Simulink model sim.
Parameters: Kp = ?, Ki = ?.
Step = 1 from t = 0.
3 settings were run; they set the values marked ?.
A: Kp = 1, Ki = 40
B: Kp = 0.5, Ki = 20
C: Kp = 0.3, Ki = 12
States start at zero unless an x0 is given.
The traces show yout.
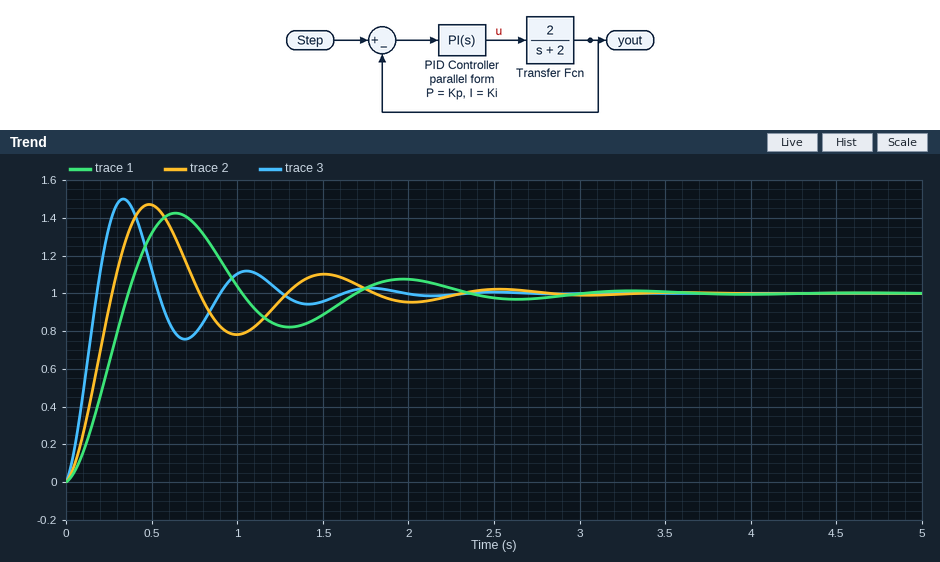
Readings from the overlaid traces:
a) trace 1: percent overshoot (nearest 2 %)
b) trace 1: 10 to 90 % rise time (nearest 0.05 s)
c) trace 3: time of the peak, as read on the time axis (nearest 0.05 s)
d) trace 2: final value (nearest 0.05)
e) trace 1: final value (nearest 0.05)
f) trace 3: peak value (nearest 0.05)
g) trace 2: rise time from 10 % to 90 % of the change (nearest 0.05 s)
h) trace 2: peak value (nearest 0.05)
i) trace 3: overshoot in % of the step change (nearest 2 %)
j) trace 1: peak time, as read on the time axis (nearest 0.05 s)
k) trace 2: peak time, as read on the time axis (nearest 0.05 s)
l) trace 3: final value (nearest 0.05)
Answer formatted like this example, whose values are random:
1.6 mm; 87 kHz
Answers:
42 %; 0.25 s; 0.35 s; 1.00; 1.00; 1.50; 0.20 s; 1.45; 50 %; 0.65 s; 0.50 s; 1.00
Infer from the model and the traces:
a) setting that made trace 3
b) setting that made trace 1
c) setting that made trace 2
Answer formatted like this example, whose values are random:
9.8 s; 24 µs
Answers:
A; C; B
